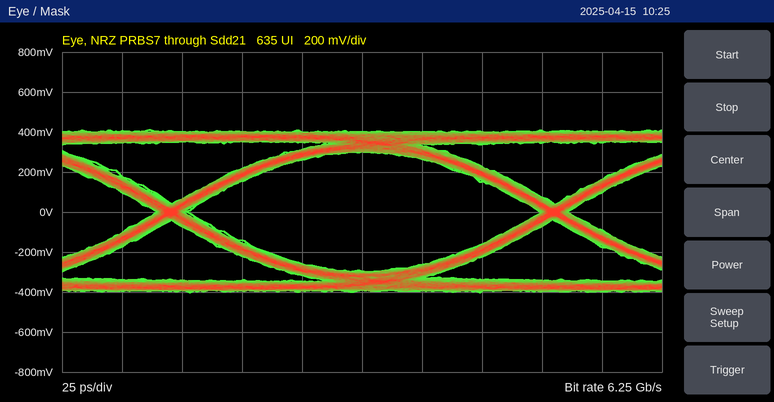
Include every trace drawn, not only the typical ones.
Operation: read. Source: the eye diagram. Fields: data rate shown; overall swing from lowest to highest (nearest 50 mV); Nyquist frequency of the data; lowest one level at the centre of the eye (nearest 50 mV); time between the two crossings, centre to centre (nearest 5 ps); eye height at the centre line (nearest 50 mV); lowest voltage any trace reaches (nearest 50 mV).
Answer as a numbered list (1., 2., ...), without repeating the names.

1. 6.25 Gb/s
2. 800 mV
3. 3.125 GHz
4. 300 mV
5. 160 ps
6. 600 mV
7. -400 mV
